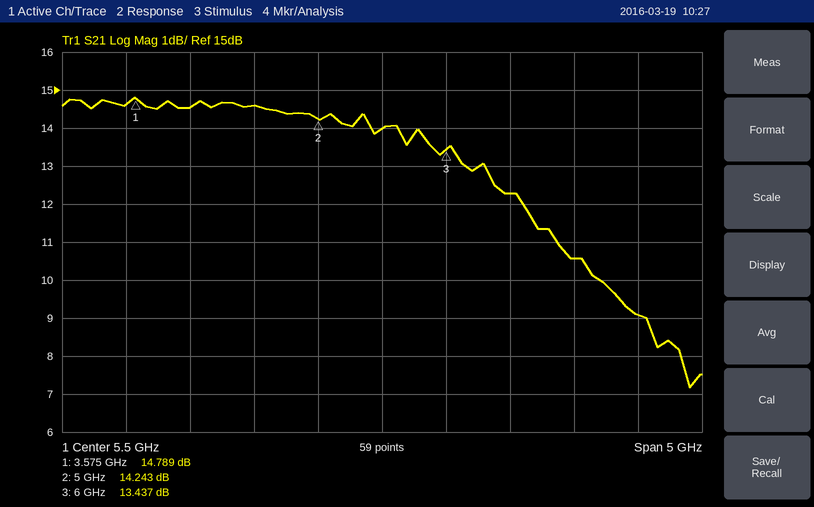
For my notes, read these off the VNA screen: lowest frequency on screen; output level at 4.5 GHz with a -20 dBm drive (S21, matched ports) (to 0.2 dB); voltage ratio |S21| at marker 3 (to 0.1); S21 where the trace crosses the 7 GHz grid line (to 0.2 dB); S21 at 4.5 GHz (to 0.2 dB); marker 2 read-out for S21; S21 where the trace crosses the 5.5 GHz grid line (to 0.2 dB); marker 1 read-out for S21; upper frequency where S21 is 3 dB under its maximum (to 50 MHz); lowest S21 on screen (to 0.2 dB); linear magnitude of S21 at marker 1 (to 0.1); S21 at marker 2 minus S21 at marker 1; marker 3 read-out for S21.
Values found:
3 GHz
-5.4 dBm
4.7
10.6 dB
14.6 dB
14.243 dB
14.0 dB
14.789 dB
6.65 GHz
7.2 dB
5.5
-0.546 dB
13.437 dB
